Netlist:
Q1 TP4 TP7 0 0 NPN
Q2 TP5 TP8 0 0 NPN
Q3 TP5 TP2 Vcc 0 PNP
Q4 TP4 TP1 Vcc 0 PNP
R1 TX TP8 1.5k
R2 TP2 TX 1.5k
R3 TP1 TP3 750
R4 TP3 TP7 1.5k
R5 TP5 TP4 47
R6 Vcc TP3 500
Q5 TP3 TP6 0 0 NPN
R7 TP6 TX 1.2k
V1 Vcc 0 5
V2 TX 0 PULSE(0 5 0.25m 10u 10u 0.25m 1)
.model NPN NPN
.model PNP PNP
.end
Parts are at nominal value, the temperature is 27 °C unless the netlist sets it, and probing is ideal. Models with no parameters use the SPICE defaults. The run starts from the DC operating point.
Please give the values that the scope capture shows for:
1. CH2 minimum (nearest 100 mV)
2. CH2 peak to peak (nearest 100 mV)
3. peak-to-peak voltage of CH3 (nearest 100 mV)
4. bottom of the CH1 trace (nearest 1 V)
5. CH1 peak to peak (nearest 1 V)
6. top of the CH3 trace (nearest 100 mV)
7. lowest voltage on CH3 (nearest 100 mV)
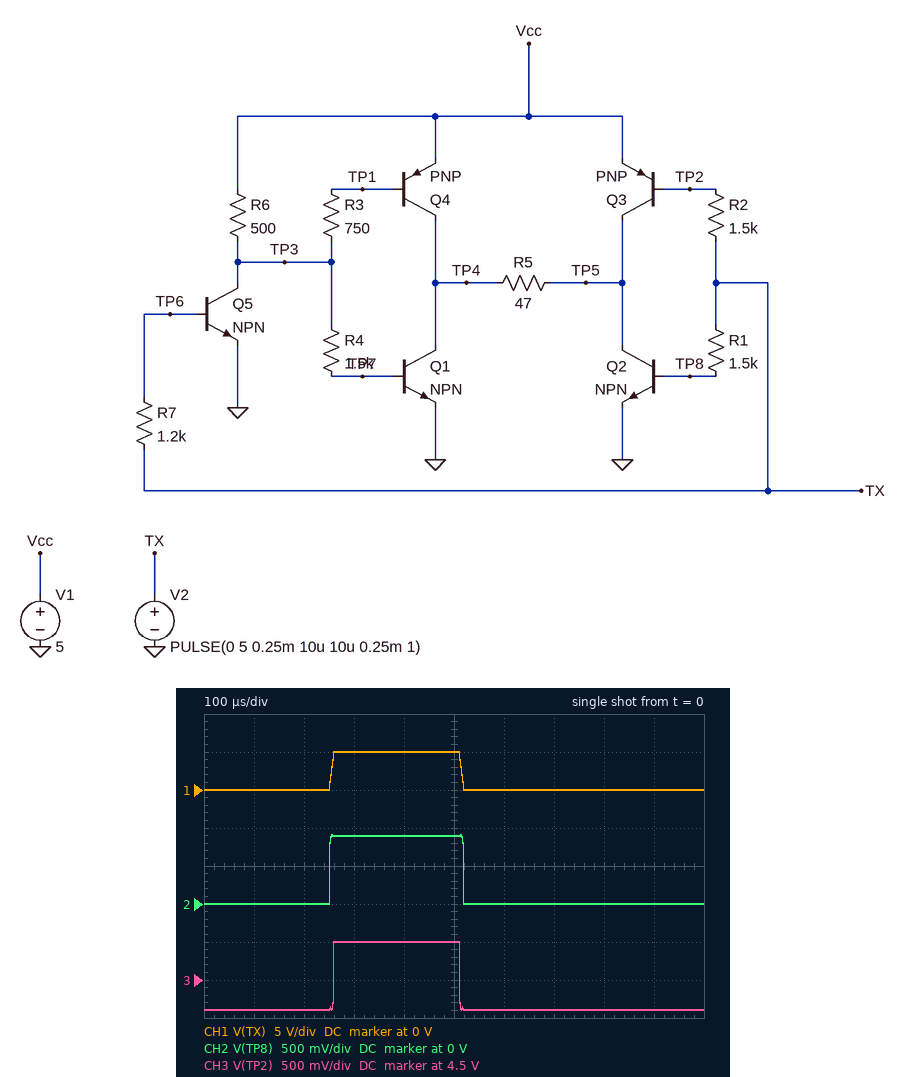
0 V
900 mV
900 mV
0 V
5 V
5.0 V
4.1 V
